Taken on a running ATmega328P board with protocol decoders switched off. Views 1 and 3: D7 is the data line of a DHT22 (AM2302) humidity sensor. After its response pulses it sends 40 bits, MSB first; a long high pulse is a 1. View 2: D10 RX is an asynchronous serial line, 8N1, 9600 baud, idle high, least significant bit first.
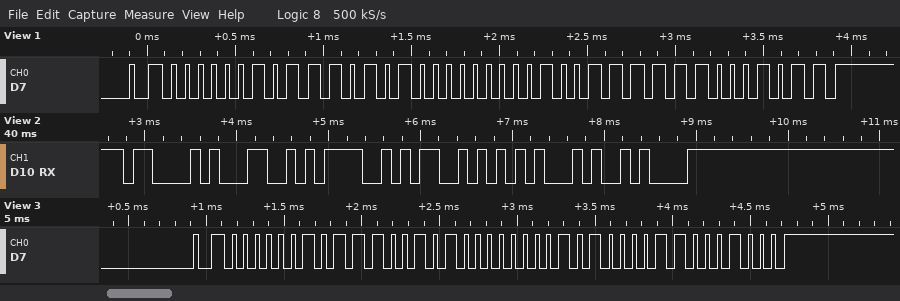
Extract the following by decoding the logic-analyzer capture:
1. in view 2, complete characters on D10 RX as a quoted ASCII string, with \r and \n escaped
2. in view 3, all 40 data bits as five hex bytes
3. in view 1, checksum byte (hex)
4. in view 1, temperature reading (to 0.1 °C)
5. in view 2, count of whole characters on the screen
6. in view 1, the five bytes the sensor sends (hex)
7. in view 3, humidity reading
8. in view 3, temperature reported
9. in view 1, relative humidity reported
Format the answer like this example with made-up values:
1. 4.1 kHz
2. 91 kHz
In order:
1. "CLOSE\n"
2. 02 E5 00 A1 88
3. 0x8B
4. 15.9 °C
5. 6
6. 02 EA 00 9F 8B
7. 74.1 %
8. 16.1 °C
9. 74.6 %
